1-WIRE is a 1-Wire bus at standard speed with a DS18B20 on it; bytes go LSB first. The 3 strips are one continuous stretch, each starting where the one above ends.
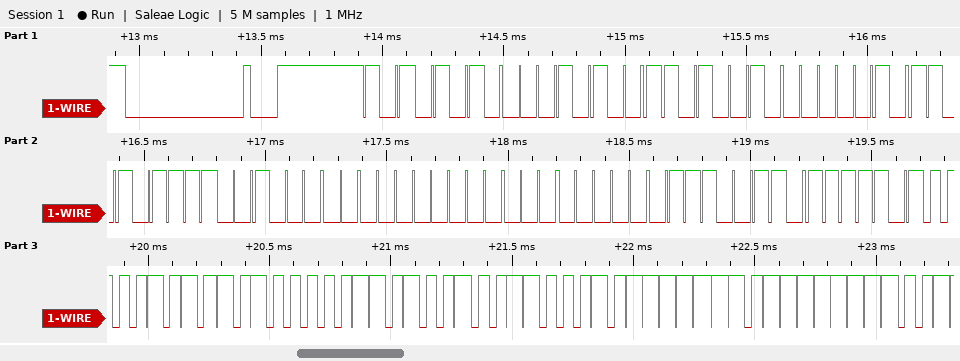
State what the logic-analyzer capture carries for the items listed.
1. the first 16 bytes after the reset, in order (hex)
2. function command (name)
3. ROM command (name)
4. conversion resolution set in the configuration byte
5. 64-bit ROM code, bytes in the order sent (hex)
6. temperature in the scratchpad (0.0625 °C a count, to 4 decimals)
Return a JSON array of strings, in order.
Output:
["55 28 4B A0 F5 04 00 00 CE BE 50 05 4B 46 7F FF", "Read Scratchpad", "Match ROM", "12 bits", "28 4B A0 F5 04 00 00 CE", "85.0000 °C"]
